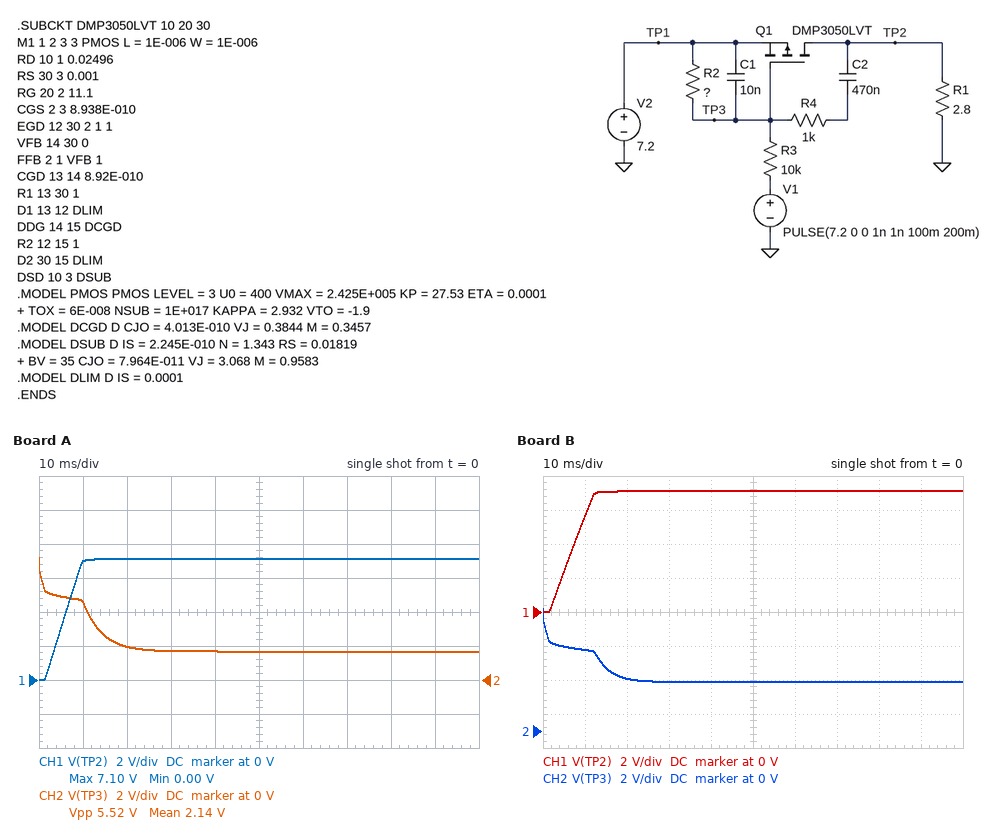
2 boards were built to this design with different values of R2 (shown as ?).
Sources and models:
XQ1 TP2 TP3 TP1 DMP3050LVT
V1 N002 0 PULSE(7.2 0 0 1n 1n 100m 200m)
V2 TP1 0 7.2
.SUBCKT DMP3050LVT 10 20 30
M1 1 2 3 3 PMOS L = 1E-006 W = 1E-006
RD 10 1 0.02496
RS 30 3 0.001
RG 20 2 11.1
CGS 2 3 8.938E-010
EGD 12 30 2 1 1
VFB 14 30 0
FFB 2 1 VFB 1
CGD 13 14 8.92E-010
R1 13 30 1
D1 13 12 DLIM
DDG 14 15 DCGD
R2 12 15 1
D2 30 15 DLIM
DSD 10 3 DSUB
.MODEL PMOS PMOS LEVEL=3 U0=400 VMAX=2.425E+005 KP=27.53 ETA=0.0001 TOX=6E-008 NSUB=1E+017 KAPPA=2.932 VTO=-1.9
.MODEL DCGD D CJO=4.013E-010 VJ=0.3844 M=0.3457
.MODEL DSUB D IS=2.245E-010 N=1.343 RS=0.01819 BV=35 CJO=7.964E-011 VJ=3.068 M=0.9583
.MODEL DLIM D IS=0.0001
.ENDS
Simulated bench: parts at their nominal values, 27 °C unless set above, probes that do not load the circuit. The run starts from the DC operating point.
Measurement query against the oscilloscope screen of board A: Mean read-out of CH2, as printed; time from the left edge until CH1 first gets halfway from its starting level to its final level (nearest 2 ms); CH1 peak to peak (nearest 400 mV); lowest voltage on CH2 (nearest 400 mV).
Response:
2.14 V
6 ms
7.2 V
1.6 V
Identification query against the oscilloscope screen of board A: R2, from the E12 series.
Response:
33 kΩ
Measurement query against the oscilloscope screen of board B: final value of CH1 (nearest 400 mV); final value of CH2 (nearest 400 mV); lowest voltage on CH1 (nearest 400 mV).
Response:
7.2 V
2.8 V
0 V
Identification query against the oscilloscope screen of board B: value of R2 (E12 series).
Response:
15 kΩ
